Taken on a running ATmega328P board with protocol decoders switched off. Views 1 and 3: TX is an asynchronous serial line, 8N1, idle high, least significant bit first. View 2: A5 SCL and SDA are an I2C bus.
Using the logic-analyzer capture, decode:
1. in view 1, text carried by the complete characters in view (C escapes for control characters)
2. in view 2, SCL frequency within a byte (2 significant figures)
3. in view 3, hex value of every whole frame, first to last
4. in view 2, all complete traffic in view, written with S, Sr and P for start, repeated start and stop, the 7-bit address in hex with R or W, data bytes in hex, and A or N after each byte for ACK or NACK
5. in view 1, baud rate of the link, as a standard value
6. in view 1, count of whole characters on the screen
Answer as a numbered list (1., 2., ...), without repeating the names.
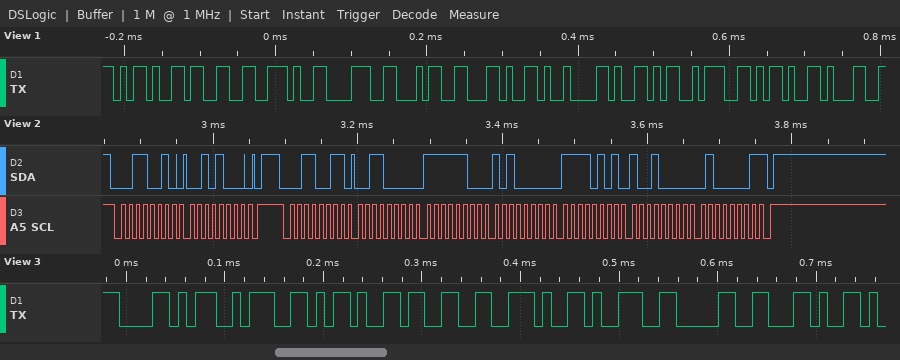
1. "-3.84,\tY:-1"
2. 100 kHz
3. 58 3A 2D 33 2E 39 30 2C
4. S 19W A 28 A P S 19R A 30 A FC A A0 A F5 A 90 A 41 N P
5. 115200 baud
6. 11
